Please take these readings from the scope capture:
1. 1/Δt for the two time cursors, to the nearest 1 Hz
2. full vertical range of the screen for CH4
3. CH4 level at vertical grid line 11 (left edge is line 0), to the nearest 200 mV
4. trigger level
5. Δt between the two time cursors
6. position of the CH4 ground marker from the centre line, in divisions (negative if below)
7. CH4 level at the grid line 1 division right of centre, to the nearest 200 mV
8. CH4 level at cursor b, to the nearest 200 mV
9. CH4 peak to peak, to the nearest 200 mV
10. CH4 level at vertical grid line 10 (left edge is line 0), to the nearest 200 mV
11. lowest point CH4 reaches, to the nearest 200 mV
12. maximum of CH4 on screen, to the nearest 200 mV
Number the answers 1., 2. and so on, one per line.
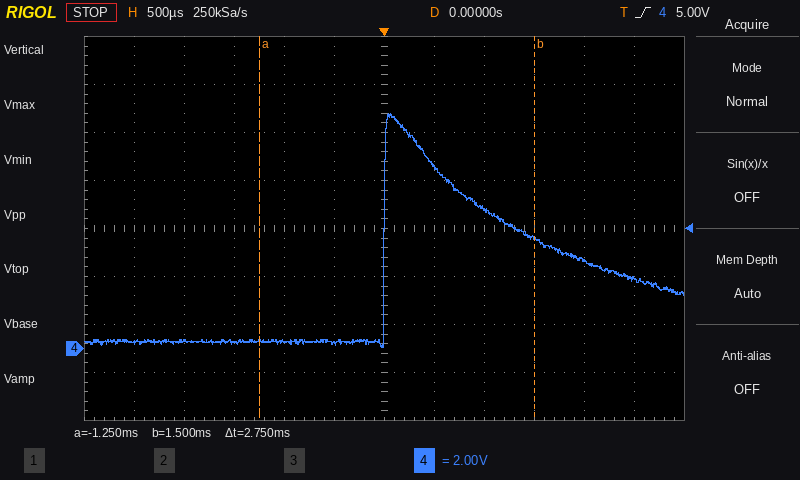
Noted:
1. 364 Hz
2. 16 V
3. 2.8 V
4. 5.00 V
5. 2.75 ms
6. -2.5 div
7. 7.6 V
8. 4.6 V
9. 9.8 V
10. 3.6 V
11. 0.0 V
12. 9.8 V
